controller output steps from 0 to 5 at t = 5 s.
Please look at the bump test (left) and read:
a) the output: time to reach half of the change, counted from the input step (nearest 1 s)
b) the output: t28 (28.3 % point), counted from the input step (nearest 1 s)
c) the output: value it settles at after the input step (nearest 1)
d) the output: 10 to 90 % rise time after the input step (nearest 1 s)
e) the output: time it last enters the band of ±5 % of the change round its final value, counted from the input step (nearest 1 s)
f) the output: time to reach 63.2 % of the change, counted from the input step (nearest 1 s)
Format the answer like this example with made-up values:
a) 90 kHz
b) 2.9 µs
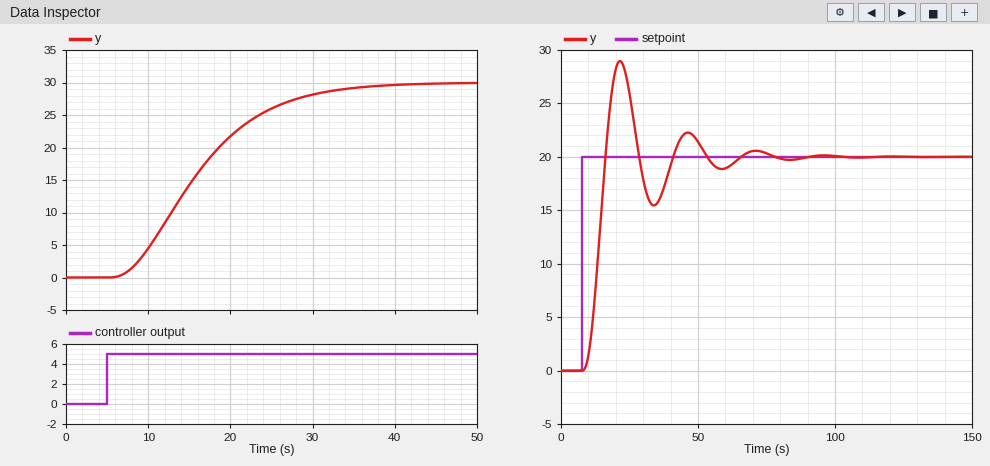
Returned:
a) 10 s
b) 7 s
c) 30
d) 18 s
e) 26 s
f) 13 s
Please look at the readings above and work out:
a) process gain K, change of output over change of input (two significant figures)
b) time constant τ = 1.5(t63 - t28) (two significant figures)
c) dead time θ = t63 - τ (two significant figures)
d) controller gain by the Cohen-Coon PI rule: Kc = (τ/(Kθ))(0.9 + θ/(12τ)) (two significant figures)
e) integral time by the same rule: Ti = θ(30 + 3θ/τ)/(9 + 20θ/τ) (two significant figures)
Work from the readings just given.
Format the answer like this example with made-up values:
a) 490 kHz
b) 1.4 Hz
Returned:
a) 6.0
b) 9.0 s
c) 4.0 s
d) 0.35
e) 7.0 s
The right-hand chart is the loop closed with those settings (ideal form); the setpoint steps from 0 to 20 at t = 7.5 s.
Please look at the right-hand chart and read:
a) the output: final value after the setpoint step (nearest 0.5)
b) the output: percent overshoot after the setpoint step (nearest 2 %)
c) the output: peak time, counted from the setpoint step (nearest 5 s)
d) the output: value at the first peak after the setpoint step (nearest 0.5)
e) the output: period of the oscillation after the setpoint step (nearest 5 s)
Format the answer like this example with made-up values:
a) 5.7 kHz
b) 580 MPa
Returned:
a) 20.0
b) 44 %
c) 15 s
d) 29.0
e) 25 s
